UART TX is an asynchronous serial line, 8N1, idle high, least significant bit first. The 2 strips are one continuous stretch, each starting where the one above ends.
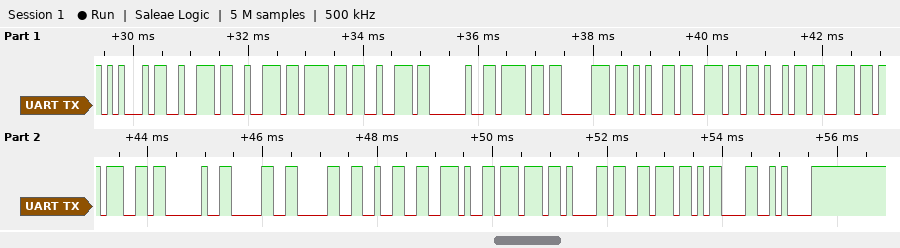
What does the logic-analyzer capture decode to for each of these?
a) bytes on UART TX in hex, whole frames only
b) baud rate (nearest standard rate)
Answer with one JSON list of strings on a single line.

["45 72 72 6F 72 20 6F 70 65 6E 69 6E 67 20 30 30 32 2E 77 61 76 0D 0A", "9600 baud"]
